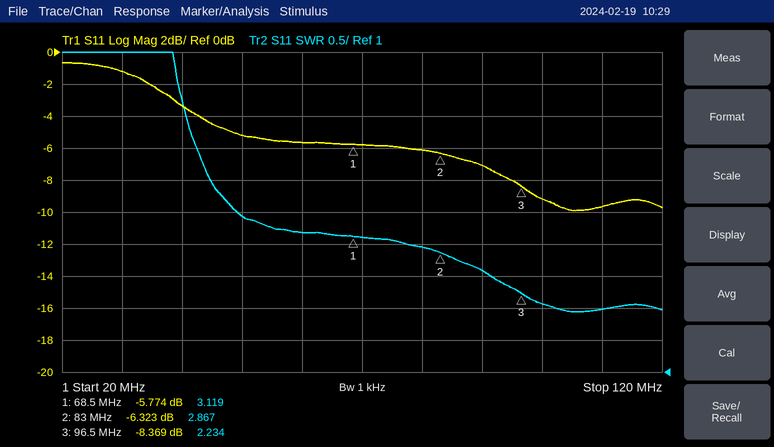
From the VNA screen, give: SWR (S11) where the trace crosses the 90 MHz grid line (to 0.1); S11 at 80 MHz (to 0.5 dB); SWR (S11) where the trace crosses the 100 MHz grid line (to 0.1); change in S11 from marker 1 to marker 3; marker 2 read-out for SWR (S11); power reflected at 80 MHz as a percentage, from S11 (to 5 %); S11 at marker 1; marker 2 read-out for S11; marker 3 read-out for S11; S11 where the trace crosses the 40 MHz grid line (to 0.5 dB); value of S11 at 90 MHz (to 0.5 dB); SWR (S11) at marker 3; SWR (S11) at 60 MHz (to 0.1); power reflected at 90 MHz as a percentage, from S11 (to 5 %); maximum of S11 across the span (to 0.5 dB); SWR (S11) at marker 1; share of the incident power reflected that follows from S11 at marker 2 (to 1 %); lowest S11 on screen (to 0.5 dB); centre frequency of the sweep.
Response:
2.6
-6.0 dB
2.1
-2.595 dB
2.867
25 %
-5.774 dB
-6.323 dB
-8.369 dB
-3.5 dB
-7.0 dB
2.234
3.2
20 %
-0.5 dB
3.119
23 %
-10.0 dB
70 MHz
